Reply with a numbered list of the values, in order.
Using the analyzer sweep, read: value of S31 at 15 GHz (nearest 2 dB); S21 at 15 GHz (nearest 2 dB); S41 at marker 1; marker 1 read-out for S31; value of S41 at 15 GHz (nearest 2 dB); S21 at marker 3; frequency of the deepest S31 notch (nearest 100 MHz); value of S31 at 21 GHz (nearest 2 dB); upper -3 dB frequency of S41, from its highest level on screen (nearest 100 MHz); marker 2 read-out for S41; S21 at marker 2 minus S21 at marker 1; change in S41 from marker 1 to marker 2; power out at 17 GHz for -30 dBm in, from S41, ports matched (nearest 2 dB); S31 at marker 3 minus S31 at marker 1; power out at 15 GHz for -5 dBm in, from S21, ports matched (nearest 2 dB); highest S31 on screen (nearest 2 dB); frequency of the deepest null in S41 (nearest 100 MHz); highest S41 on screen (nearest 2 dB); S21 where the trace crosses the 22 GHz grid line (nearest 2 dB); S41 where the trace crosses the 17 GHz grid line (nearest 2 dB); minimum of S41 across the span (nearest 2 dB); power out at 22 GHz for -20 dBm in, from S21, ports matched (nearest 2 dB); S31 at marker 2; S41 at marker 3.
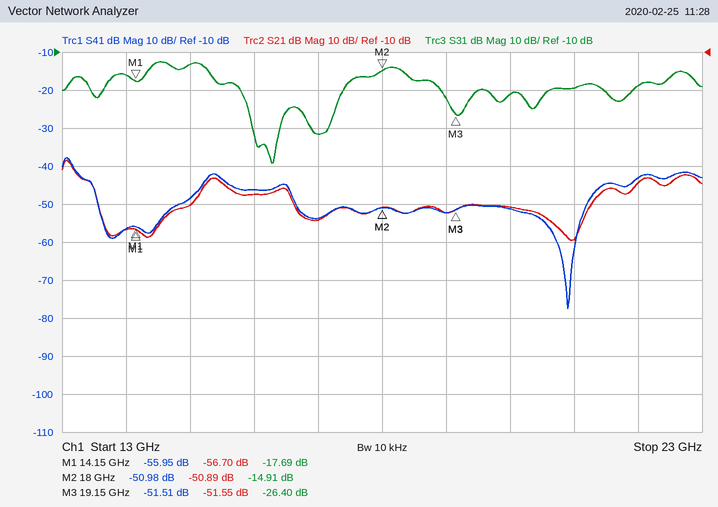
1. -14 dB
2. -50 dB
3. -55.95 dB
4. -17.69 dB
5. -48 dB
6. -51.55 dB
7. 16.3 GHz
8. -20 dB
9. 13.2 GHz
10. -50.98 dB
11. 5.81 dB
12. 4.97 dB
13. -84 dBm
14. -8.71 dB
15. -56 dBm
16. -12 dB
17. 20.9 GHz
18. -38 dB
19. -44 dB
20. -54 dB
21. -78 dB
22. -64 dBm
23. -14.91 dB
24. -51.51 dB
